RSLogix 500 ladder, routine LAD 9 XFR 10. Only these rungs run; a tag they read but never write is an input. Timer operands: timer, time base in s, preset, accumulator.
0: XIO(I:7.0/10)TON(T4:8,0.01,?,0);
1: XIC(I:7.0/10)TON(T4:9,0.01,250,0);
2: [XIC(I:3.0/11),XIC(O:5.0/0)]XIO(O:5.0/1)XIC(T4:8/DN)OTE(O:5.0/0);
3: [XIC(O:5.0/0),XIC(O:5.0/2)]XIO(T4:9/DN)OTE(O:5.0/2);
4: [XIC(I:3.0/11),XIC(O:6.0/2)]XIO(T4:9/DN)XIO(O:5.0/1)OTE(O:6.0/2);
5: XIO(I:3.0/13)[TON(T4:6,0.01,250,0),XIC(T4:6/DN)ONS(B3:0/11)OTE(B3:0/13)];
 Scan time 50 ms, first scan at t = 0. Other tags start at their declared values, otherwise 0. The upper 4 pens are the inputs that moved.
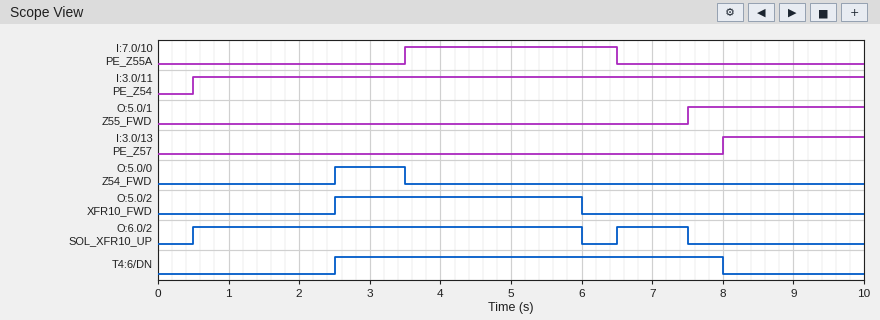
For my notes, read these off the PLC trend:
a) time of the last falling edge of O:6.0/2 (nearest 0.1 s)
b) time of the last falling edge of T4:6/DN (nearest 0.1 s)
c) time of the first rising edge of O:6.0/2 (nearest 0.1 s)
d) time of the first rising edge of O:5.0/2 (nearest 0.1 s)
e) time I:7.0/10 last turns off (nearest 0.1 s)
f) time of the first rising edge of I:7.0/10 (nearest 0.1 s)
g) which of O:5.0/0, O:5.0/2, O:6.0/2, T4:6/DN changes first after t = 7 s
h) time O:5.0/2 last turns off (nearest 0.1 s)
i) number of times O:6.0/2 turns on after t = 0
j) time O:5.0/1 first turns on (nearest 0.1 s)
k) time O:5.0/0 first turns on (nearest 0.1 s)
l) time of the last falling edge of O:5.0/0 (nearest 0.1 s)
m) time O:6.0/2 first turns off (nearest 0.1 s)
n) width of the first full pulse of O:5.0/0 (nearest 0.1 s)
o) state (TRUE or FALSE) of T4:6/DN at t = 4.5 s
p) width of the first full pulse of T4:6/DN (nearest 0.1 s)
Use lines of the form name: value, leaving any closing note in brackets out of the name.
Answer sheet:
time of the last falling edge of O:6.0/2: 7.5 s
time of the last falling edge of T4:6/DN: 8.0 s
time of the first rising edge of O:6.0/2: 0.5 s
time of the first rising edge of O:5.0/2: 2.5 s
time I:7.0/10 last turns off: 6.5 s
time of the first rising edge of I:7.0/10: 3.5 s
which of O:5.0/0, O:5.0/2, O:6.0/2, T4:6/DN changes first after t = 7 s: O:6.0/2
time O:5.0/2 last turns off: 6.0 s
number of times O:6.0/2 turns on after t = 0: 2
time O:5.0/1 first turns on: 7.5 s
time O:5.0/0 first turns on: 2.5 s
time of the last falling edge of O:5.0/0: 3.5 s
time O:6.0/2 first turns off: 6.0 s
width of the first full pulse of O:5.0/0: 1.0 s
state (TRUE or FALSE) of T4:6/DN at t = 4.5 s: TRUE
width of the first full pulse of T4:6/DN: 5.5 s
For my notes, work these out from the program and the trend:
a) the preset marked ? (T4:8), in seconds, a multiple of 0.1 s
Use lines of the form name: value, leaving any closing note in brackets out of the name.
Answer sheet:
the preset marked ? (T4:8), in seconds, a multiple of 0.1 s: 2.5 s
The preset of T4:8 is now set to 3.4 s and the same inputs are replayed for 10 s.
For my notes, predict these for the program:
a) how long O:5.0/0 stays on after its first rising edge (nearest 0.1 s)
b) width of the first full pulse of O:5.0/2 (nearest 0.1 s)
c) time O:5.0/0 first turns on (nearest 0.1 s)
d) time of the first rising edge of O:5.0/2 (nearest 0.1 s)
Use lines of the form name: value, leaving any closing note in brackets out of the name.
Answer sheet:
how long O:5.0/0 stays on after its first rising edge: 0.1 s
width of the first full pulse of O:5.0/2: 2.6 s
time O:5.0/0 first turns on: 3.4 s
time of the first rising edge of O:5.0/2: 3.4 s
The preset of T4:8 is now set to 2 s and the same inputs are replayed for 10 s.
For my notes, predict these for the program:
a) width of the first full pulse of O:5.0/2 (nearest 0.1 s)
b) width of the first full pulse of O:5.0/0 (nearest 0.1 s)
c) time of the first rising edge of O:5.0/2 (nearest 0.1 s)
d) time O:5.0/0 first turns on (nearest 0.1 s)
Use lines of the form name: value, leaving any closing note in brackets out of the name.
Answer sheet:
width of the first full pulse of O:5.0/2: 4.0 s
width of the first full pulse of O:5.0/0: 1.5 s
time of the first rising edge of O:5.0/2: 2.0 s
time O:5.0/0 first turns on: 2.0 s
